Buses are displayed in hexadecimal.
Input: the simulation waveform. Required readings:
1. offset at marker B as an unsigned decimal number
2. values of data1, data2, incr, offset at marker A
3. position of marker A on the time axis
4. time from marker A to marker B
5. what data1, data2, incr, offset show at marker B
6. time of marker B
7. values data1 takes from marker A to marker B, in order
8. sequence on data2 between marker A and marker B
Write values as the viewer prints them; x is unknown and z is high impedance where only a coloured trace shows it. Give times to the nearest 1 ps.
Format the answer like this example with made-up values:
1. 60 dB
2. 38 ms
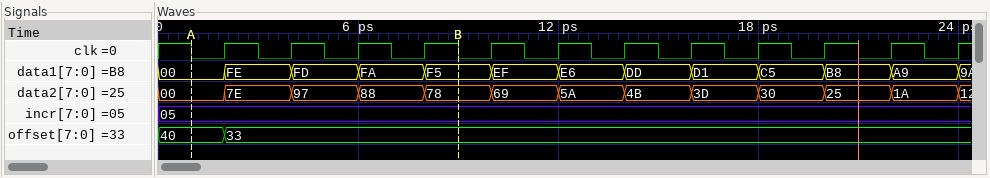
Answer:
1. 51
2. data1=00, data2=00, incr=05, offset=40
3. 1 ps
4. 8 ps
5. data1=F5, data2=78, incr=05, offset=33
6. 9 ps
7. 00, FE, FD, FA, F5
8. 00, 7E, 97, 88, 78
